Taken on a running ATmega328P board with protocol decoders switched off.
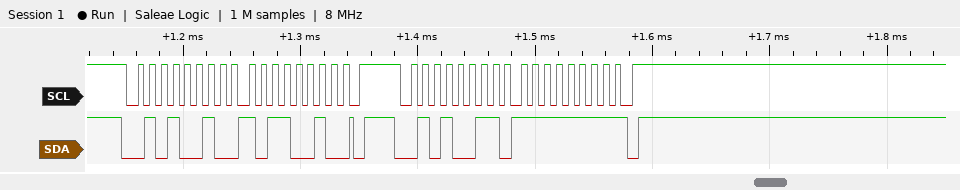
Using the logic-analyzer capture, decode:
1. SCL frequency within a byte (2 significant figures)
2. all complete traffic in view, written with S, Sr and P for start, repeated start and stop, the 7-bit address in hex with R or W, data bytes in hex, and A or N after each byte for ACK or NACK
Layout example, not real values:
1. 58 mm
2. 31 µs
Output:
1. 100 kHz
2. S 29W A B2 A P S 29R A FF N P
